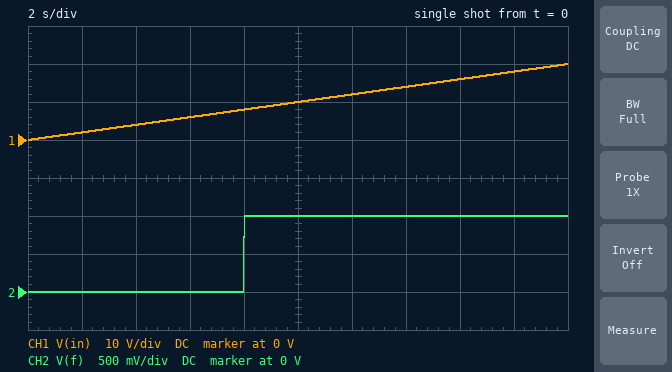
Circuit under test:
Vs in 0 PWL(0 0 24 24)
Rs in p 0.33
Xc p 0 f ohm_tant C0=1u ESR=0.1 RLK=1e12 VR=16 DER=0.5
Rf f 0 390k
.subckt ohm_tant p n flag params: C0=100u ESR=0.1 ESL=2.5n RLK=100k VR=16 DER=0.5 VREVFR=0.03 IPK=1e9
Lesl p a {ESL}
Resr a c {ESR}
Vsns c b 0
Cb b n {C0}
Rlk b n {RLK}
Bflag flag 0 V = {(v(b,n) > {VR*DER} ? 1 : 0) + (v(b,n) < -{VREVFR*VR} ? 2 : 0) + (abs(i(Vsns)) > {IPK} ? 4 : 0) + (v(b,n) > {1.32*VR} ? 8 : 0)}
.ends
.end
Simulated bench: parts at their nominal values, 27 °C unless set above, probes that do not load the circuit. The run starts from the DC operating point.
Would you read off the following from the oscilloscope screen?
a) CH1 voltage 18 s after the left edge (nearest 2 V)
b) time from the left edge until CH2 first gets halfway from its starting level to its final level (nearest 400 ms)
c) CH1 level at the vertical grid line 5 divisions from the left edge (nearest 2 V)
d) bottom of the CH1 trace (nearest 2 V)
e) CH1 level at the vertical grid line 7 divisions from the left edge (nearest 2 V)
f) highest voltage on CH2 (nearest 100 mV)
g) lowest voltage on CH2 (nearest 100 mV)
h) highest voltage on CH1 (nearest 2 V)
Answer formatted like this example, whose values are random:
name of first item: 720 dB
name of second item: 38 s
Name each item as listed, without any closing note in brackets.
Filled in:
CH1 voltage 18 s after the left edge: 18 V
time from the left edge until CH2 first gets halfway from its starting level to its final level: 8.0 s
CH1 level at the vertical grid line 5 divisions from the left edge: 10 V
bottom of the CH1 trace: 0 V
CH1 level at the vertical grid line 7 divisions from the left edge: 14 V
highest voltage on CH2: 1.0 V
lowest voltage on CH2: 0 V
highest voltage on CH1: 20 V
